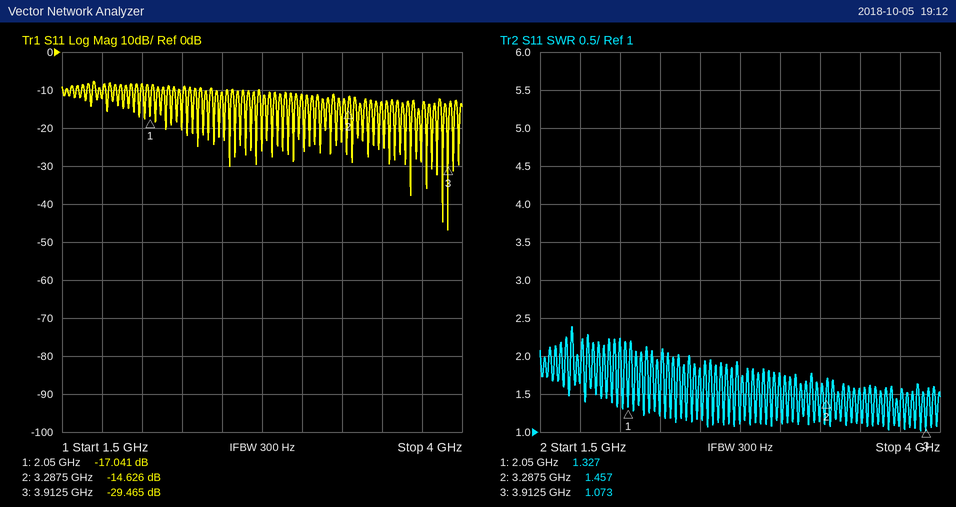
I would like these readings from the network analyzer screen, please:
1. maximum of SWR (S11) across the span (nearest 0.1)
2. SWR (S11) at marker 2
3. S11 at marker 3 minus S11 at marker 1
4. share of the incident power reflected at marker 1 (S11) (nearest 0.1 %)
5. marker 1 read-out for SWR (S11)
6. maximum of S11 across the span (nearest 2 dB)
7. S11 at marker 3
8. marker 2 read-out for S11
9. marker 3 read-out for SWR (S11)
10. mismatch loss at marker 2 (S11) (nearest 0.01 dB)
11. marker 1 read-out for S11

2.4
1.457
-12.424 dB
2.0 %
1.327
-8 dB
-29.465 dB
-14.626 dB
1.073
0.15 dB
-17.041 dB
